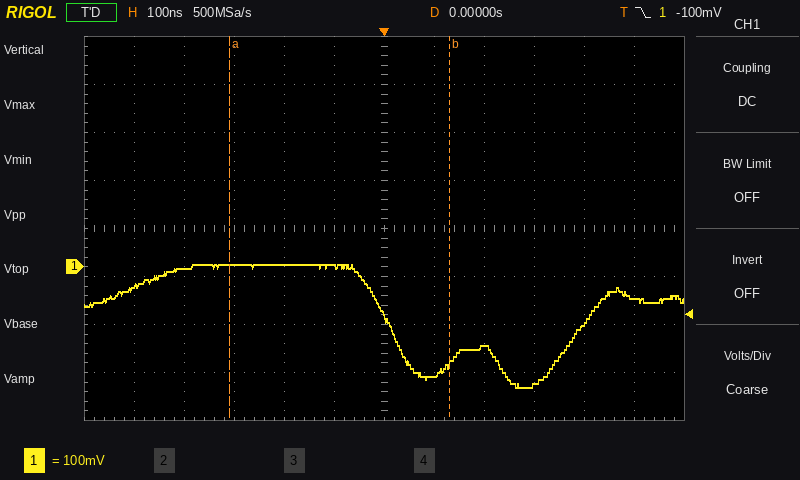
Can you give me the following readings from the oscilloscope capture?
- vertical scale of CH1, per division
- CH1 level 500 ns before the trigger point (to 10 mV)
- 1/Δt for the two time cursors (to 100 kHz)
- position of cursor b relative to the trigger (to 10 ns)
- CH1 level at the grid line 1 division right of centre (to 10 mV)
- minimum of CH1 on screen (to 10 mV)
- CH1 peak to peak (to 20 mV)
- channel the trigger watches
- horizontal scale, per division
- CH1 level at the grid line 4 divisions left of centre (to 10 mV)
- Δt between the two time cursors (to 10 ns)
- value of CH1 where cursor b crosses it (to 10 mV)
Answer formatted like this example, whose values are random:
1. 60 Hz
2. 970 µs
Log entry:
1. 100 mV
2. -40 mV
3. 2.3 MHz
4. +130 ns
5. -230 mV
6. -250 mV
7. 260 mV
8. CH1
9. 100 ns
10. 0 mV
11. 440 ns
12. -200 mV
